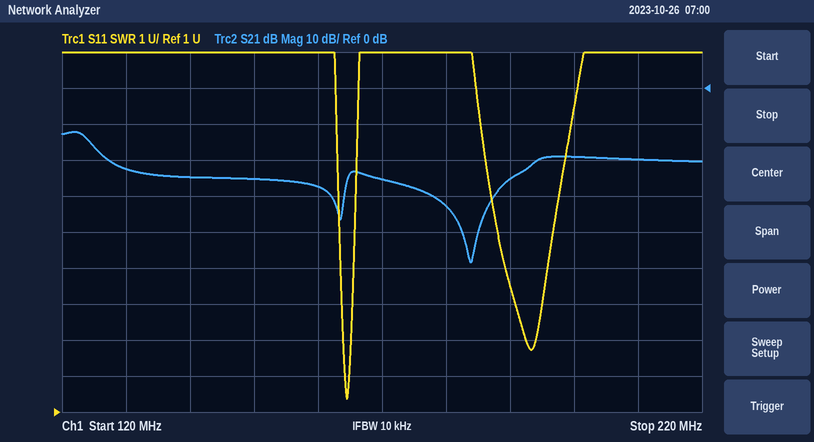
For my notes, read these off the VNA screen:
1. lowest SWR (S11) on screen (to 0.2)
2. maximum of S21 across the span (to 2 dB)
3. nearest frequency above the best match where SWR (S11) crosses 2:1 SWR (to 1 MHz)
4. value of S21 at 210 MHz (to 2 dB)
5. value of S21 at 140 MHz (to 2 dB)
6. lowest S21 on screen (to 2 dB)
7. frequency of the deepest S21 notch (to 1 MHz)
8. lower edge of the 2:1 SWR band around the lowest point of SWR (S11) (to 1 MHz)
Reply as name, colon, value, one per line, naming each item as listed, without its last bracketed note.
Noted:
lowest SWR (S11) on screen: 1.4
maximum of S21 across the span: -12 dB
nearest frequency above the best match where SWR (S11) crosses 2:1 SWR: 165 MHz
value of S21 at 210 MHz: -20 dB
value of S21 at 140 MHz: -24 dB
lowest S21 on screen: -48 dB
frequency of the deepest S21 notch: 184 MHz
lower edge of the 2:1 SWR band around the lowest point of SWR (S11): 164 MHz
